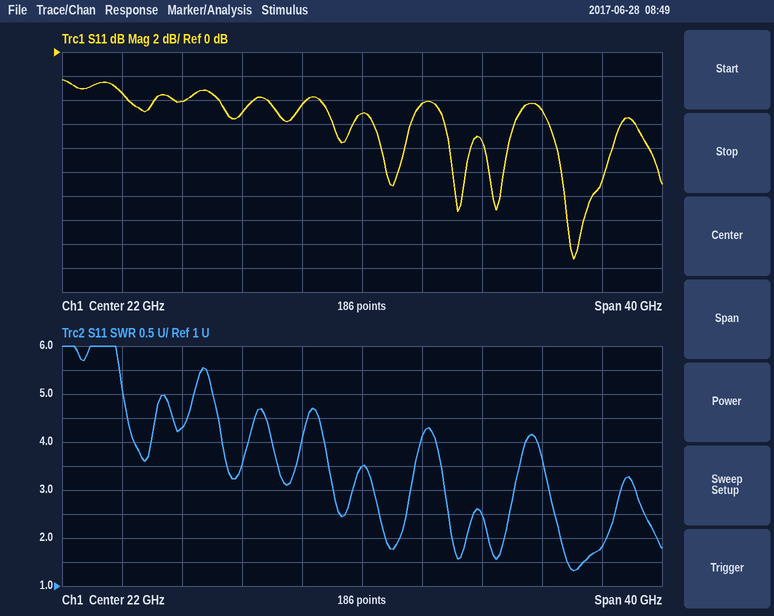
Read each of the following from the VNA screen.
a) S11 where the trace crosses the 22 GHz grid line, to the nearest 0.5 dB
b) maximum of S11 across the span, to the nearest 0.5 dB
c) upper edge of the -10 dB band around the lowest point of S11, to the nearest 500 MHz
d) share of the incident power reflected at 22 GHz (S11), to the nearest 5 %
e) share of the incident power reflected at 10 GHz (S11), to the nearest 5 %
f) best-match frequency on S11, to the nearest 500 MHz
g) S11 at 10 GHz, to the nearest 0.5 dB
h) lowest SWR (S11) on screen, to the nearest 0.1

-5.0 dB
-2.5 dB
38.0 GHz
30 %
40 %
36.0 GHz
-4.0 dB
1.3
